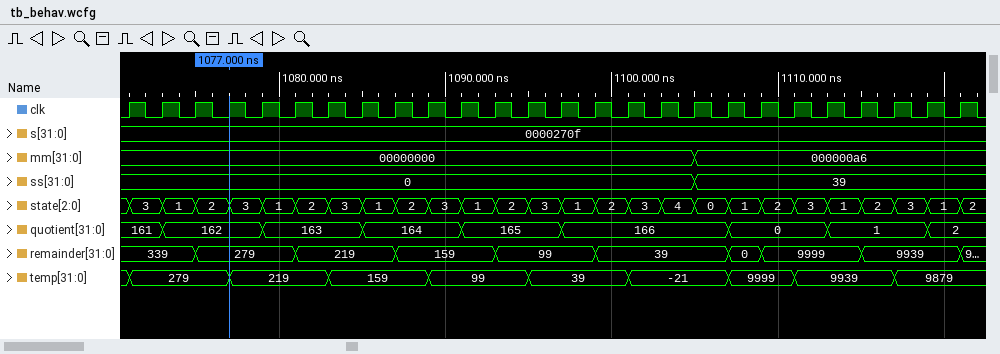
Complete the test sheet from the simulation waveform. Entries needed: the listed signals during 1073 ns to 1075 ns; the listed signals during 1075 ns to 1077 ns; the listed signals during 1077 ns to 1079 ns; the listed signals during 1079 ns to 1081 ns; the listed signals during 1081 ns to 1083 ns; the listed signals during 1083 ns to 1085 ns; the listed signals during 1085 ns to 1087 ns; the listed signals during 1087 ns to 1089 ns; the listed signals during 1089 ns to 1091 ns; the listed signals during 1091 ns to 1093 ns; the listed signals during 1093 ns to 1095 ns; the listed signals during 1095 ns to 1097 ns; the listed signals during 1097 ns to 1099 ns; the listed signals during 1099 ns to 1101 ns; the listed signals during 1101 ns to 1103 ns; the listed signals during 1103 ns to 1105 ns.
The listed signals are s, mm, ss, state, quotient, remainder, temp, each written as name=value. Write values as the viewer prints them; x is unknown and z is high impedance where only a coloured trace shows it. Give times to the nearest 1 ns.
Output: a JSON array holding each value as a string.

["s=0000270f, mm=00000000, ss=0, state=1, quotient=162, remainder=339, temp=279", "s=0000270f, mm=00000000, ss=0, state=2, quotient=162, remainder=279, temp=279", "s=0000270f, mm=00000000, ss=0, state=3, quotient=162, remainder=279, temp=219", "s=0000270f, mm=00000000, ss=0, state=1, quotient=163, remainder=279, temp=219", "s=0000270f, mm=00000000, ss=0, state=2, quotient=163, remainder=219, temp=219", "s=0000270f, mm=00000000, ss=0, state=3, quotient=163, remainder=219, temp=159", "s=0000270f, mm=00000000, ss=0, state=1, quotient=164, remainder=219, temp=159", "s=0000270f, mm=00000000, ss=0, state=2, quotient=164, remainder=159, temp=159", "s=0000270f, mm=00000000, ss=0, state=3, quotient=164, remainder=159, temp=99", "s=0000270f, mm=00000000, ss=0, state=1, quotient=165, remainder=159, temp=99", "s=0000270f, mm=00000000, ss=0, state=2, quotient=165, remainder=99, temp=99", "s=0000270f, mm=00000000, ss=0, state=3, quotient=165, remainder=99, temp=39", "s=0000270f, mm=00000000, ss=0, state=1, quotient=166, remainder=99, temp=39", "s=0000270f, mm=00000000, ss=0, state=2, quotient=166, remainder=39, temp=39", "s=0000270f, mm=00000000, ss=0, state=3, quotient=166, remainder=39, temp=-21", "s=0000270f, mm=00000000, ss=0, state=4, quotient=166, remainder=39, temp=-21"]
